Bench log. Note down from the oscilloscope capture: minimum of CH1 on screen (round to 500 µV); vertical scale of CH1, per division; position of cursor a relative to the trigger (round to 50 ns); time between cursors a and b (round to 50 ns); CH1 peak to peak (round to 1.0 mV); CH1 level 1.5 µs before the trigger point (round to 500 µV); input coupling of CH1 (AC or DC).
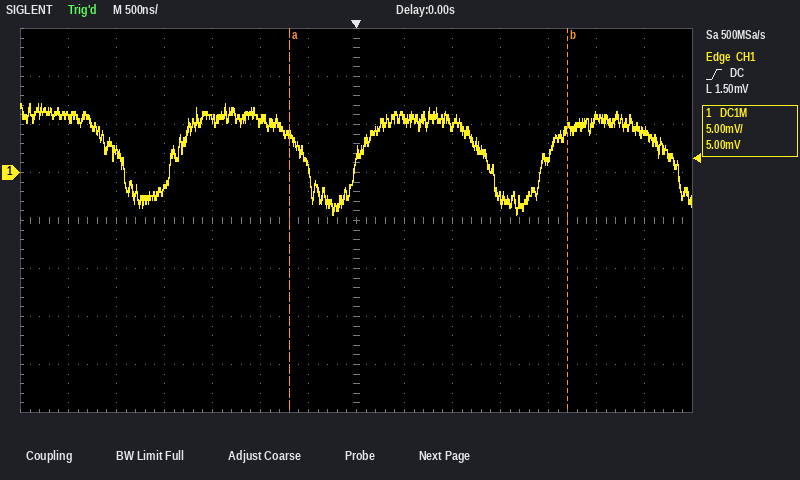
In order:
-4.5 mV
5 mV
-700 ns
2.90 µs
12.0 mV
5.5 mV
DC
